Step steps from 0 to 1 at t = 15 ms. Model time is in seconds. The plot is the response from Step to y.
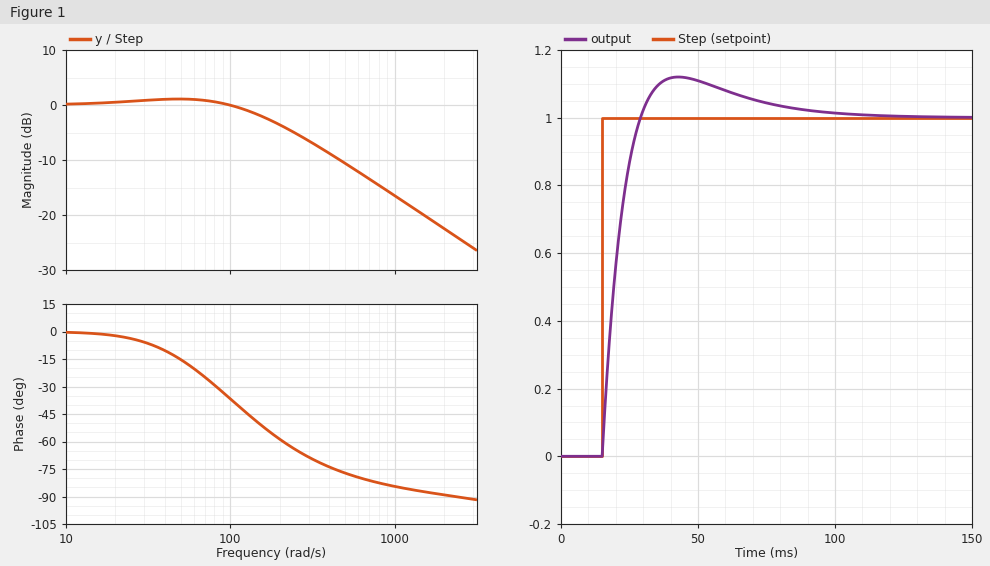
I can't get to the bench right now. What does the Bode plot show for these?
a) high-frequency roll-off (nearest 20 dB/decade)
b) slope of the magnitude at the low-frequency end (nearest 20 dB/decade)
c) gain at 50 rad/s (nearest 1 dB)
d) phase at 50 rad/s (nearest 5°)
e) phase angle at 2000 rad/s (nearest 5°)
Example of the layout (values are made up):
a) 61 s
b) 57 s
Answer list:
a) -20 dB/decade
b) 0 dB/decade
c) 1 dB
d) -15°
e) -90°
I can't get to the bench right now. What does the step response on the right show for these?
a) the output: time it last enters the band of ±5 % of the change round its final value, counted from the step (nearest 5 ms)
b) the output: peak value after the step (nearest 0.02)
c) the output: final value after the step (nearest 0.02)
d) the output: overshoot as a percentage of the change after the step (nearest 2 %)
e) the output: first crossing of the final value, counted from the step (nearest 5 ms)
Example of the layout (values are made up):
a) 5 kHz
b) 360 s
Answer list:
a) 55 ms
b) 1.12
c) 1.00
d) 12 %
e) 15 ms
